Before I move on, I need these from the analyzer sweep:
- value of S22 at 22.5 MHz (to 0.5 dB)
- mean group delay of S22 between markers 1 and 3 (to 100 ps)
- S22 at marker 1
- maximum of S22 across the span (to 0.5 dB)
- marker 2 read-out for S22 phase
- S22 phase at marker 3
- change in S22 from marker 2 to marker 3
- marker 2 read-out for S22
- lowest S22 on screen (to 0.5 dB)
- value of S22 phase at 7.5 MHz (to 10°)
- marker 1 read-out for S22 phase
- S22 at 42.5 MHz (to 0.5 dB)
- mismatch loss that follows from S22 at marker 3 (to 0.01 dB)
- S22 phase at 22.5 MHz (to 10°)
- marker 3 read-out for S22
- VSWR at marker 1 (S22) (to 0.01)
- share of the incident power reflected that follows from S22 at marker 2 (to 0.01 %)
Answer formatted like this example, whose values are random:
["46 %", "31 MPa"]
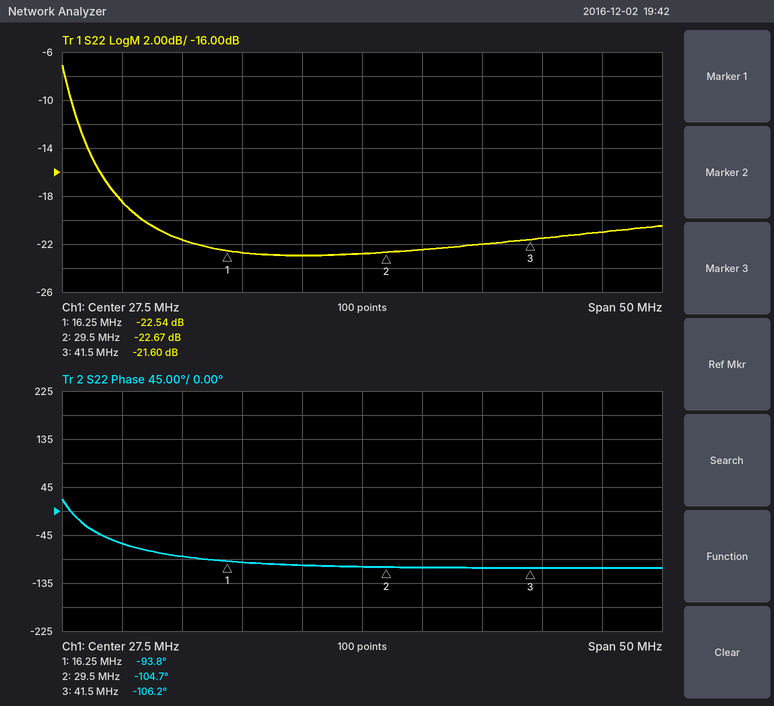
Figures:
["-23.0 dB", "1.4 ns", "-22.54 dB", "-7.0 dB", "-104.7°", "-106.2°", "1.07 dB", "-22.67 dB", "-23.0 dB", "-60°", "-93.8°", "-21.5 dB", "0.03 dB", "-100°", "-21.60 dB", "1.16", "0.54 %"]
